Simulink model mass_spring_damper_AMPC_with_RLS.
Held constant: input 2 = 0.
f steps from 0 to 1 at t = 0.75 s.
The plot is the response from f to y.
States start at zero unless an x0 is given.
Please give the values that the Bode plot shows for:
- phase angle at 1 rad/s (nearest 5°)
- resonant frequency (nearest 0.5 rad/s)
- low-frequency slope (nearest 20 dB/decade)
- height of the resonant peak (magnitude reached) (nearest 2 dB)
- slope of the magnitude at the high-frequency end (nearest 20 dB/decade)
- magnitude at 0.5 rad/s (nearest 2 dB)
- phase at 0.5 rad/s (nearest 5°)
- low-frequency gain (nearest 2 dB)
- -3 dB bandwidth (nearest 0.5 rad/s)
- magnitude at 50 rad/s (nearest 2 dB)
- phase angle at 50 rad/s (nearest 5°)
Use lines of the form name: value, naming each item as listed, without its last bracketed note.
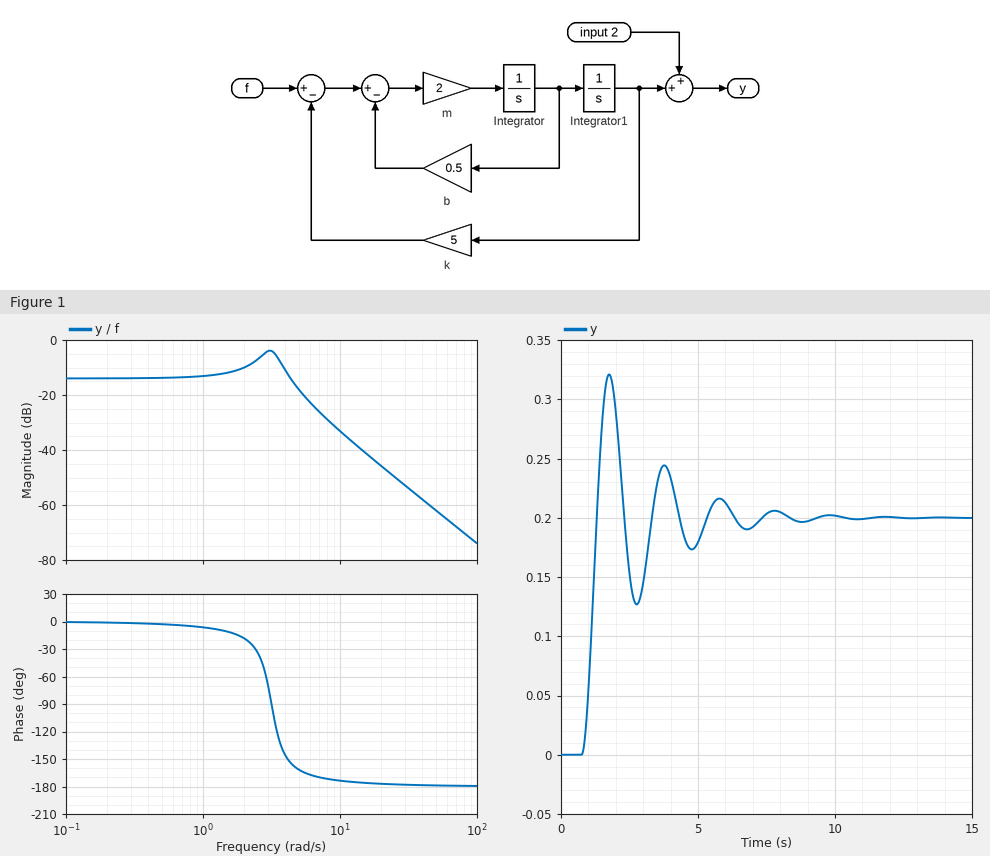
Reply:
phase angle at 1 rad/s: -5°
resonant frequency: 3.0 rad/s
low-frequency slope: 0 dB/decade
height of the resonant peak (magnitude reached): -4 dB
slope of the magnitude at the high-frequency end: -40 dB/decade
magnitude at 0.5 rad/s: -14 dB
phase at 0.5 rad/s: -5°
low-frequency gain: -14 dB
-3 dB bandwidth: 5.0 rad/s
magnitude at 50 rad/s: -62 dB
phase angle at 50 rad/s: -180°
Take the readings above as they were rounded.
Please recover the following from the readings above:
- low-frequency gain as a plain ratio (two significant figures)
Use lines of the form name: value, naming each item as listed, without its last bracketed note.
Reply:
low-frequency gain as a plain ratio: 0.20
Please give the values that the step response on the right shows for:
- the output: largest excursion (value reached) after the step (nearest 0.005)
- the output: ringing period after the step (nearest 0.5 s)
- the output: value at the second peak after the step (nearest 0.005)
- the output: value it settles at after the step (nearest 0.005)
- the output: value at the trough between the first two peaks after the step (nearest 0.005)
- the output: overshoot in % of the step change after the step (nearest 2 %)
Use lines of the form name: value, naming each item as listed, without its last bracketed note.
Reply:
the output: largest excursion (value reached) after the step: 0.320
the output: ringing period after the step: 2.0 s
the output: value at the second peak after the step: 0.245
the output: value it settles at after the step: 0.200
the output: value at the trough between the first two peaks after the step: 0.125
the output: overshoot in % of the step change after the step: 60 %
